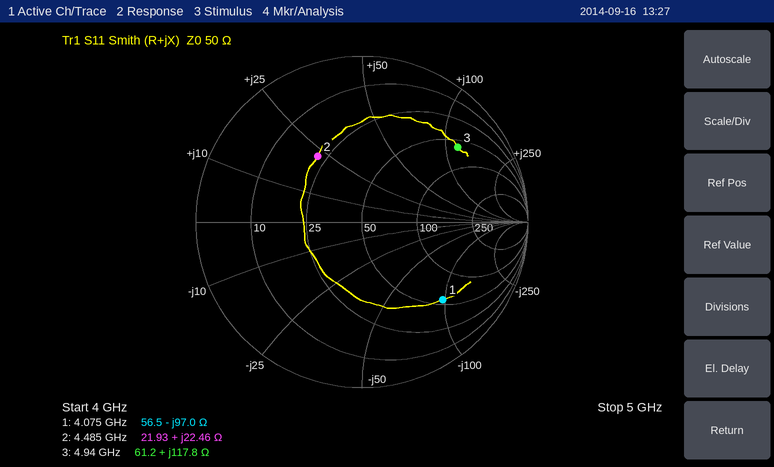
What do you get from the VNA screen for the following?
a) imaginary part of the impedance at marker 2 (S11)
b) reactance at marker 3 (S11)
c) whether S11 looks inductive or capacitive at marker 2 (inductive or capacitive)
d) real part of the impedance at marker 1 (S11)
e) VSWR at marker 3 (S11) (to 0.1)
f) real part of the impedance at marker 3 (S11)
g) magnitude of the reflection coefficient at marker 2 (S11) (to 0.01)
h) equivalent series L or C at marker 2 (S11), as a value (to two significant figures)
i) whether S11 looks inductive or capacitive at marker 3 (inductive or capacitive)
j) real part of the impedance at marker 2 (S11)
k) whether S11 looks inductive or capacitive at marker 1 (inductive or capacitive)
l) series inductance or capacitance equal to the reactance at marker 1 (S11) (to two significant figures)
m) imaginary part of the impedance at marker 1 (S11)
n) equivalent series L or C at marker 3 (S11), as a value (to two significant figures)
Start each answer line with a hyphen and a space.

- +22.46 Ω
- +117.8 Ω
- inductive
- 56.5 Ω
- 6.4
- 61.2 Ω
- 0.48
- 800 pH
- inductive
- 21.93 Ω
- capacitive
- 400 fF
- -97.0 Ω
- 3.8 nH
